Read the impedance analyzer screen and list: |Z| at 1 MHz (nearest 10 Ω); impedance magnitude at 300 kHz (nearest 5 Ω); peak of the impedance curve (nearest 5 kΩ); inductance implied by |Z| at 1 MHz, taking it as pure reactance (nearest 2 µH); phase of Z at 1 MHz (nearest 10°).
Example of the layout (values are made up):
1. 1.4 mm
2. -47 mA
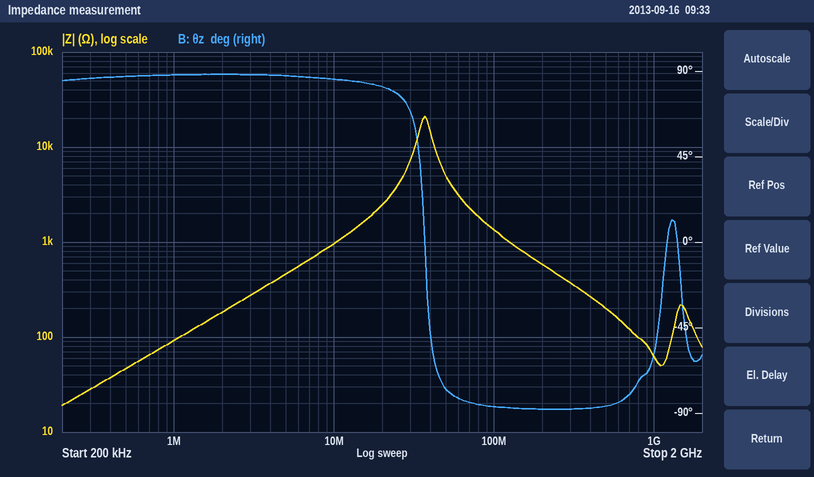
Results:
1. 90 Ω
2. 30 Ω
3. 20 kΩ
4. 14 µH
5. 90°
